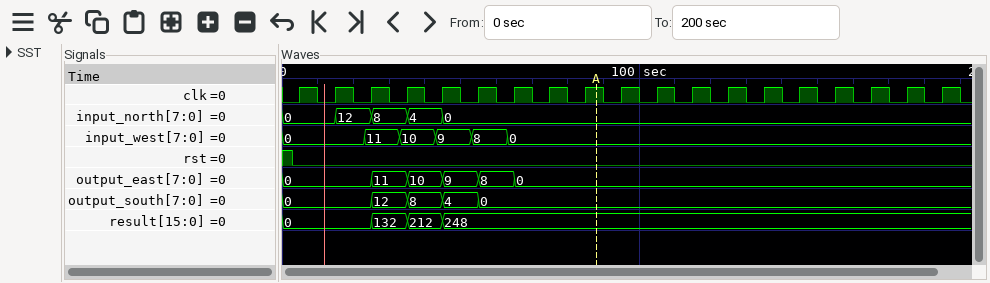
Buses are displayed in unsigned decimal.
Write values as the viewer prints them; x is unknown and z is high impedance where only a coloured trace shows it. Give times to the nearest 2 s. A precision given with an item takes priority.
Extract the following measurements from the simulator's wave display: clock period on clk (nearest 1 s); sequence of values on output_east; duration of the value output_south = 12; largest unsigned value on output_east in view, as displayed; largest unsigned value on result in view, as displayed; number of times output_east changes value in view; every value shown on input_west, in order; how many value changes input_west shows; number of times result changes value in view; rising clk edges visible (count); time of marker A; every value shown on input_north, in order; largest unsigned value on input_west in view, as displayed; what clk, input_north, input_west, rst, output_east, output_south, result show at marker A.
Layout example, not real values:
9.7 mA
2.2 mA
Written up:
10 s
0, 11, 10, 9, 8, 0
10 s
11
248
5
0, 11, 10, 9, 8, 0
5
3
19
88 s
0, 12, 8, 4, 0
11
clk=1, input_north=0, input_west=0, rst=0, output_east=0, output_south=0, result=248
